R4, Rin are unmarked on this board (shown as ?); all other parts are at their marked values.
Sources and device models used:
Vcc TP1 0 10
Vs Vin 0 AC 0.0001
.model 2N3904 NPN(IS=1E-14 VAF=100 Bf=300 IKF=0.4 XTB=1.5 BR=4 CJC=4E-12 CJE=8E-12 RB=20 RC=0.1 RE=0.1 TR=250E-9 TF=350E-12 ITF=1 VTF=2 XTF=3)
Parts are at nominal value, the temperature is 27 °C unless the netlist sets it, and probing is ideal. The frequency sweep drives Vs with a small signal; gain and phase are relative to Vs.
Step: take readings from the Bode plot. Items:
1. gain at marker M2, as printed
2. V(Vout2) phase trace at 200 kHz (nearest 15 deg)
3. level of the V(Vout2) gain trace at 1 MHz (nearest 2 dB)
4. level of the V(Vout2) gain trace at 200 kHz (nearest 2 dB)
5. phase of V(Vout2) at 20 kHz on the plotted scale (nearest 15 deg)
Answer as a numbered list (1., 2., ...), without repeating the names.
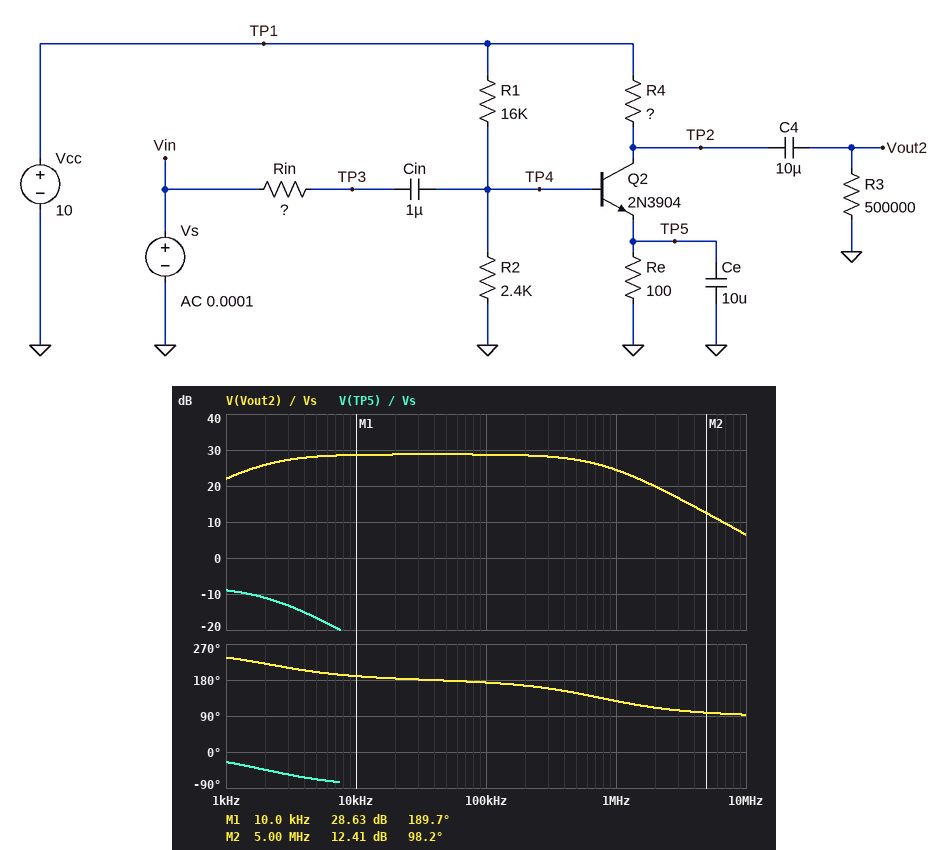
1. 12.41 dB
2. 165 deg
3. 24 dB
4. 28 dB
5. 180 deg
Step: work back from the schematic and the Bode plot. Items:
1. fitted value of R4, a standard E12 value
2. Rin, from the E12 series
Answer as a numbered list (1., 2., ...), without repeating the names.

1. 560 Ω
2. 2.7 kΩ
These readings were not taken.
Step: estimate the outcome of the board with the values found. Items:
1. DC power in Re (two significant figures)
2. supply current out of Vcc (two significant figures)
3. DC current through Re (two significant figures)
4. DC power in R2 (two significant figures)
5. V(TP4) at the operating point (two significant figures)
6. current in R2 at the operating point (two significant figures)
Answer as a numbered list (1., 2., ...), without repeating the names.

1. 3.2 mW
2. 6.2 mA
3. 5.7 mA
4. 670 µW
5. 1.3 V
6. 530 µA
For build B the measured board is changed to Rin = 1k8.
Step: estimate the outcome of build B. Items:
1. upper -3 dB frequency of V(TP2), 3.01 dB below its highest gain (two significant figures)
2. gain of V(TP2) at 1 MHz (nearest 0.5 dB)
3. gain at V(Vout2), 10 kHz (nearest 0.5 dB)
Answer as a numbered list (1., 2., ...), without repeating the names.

1. 860 kHz
2. 27.5 dB
3. 31.0 dB
